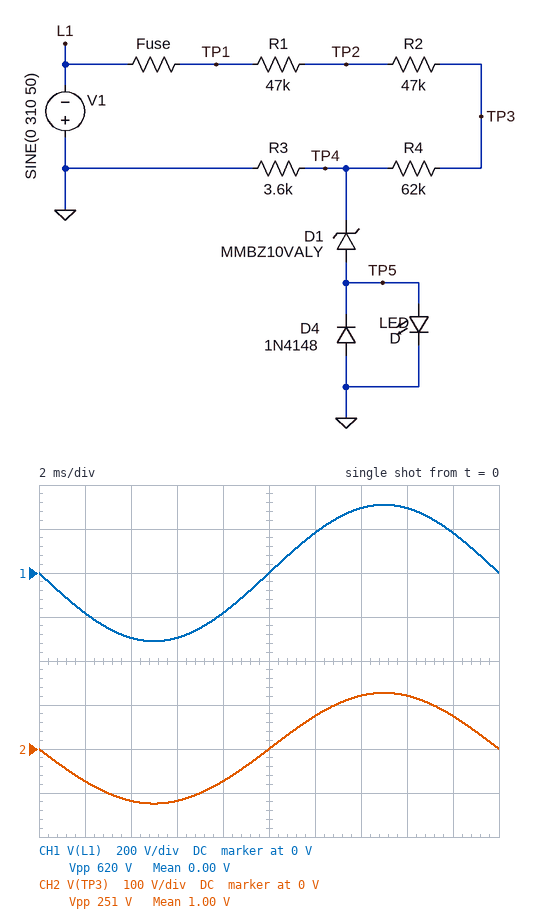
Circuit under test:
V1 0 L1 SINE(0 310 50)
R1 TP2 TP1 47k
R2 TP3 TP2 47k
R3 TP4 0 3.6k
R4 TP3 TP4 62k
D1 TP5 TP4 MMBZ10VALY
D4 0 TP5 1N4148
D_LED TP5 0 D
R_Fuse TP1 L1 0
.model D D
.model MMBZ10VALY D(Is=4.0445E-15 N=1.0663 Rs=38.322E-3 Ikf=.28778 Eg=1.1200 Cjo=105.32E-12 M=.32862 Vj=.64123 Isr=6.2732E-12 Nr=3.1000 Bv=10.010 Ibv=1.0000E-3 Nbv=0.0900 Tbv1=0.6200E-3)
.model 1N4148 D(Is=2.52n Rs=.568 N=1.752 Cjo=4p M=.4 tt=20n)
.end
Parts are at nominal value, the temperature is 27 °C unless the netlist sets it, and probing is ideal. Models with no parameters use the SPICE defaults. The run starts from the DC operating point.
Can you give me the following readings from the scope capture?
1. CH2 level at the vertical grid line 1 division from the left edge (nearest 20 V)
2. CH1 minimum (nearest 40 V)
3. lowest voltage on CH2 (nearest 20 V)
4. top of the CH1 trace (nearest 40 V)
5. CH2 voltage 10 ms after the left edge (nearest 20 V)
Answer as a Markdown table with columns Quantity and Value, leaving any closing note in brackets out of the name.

| Quantity | Value |
|---|---|
| CH2 level at the vertical grid line 1 division from the left edge | -80 V |
| CH1 minimum | -320 V |
| lowest voltage on CH2 | -120 V |
| top of the CH1 trace | 320 V |
| CH2 voltage 10 ms after the left edge | 0 V |
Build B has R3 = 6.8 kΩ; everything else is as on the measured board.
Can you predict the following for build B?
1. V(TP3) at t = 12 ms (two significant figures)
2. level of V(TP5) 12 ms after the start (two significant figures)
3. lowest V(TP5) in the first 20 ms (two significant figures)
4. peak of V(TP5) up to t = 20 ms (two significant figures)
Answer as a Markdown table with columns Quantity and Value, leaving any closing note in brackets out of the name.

| Quantity | Value |
|---|---|
| V(TP3) at t = 12 ms | 77 V |
| level of V(TP5) 12 ms after the start | 430 mV |
| lowest V(TP5) in the first 20 ms | -610 mV |
| peak of V(TP5) up to t = 20 ms | 630 mV |
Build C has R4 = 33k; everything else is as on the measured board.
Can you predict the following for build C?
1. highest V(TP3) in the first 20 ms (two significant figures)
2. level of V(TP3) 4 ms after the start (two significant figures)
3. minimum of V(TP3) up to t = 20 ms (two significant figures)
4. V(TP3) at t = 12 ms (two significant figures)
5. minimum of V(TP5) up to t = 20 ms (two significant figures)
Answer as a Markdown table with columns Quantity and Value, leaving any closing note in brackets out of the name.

| Quantity | Value |
|---|---|
| highest V(TP3) in the first 20 ms | 87 V |
| level of V(TP3) 4 ms after the start | -78 V |
| minimum of V(TP3) up to t = 20 ms | -82 V |
| V(TP3) at t = 12 ms | 51 V |
| minimum of V(TP5) up to t = 20 ms | -620 mV |
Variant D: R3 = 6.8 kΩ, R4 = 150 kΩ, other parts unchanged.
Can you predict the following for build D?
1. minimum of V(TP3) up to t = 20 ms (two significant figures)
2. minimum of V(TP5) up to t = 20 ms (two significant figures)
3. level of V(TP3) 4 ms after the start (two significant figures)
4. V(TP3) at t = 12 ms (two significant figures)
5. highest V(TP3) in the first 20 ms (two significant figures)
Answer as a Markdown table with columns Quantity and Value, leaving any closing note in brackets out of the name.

| Quantity | Value |
|---|---|
| minimum of V(TP3) up to t = 20 ms | -190 V |
| minimum of V(TP5) up to t = 20 ms | -590 mV |
| level of V(TP3) 4 ms after the start | -180 V |
| V(TP3) at t = 12 ms | 110 V |
| highest V(TP3) in the first 20 ms | 190 V |
